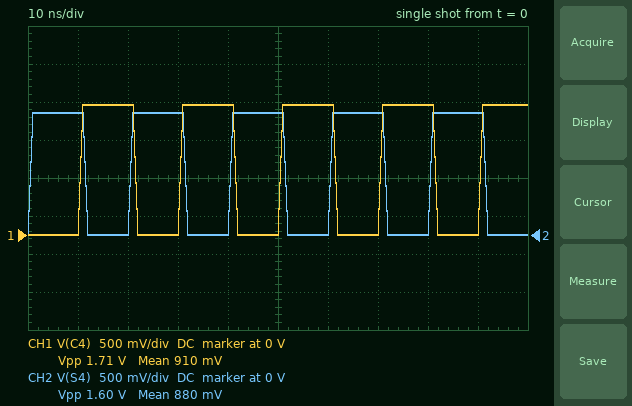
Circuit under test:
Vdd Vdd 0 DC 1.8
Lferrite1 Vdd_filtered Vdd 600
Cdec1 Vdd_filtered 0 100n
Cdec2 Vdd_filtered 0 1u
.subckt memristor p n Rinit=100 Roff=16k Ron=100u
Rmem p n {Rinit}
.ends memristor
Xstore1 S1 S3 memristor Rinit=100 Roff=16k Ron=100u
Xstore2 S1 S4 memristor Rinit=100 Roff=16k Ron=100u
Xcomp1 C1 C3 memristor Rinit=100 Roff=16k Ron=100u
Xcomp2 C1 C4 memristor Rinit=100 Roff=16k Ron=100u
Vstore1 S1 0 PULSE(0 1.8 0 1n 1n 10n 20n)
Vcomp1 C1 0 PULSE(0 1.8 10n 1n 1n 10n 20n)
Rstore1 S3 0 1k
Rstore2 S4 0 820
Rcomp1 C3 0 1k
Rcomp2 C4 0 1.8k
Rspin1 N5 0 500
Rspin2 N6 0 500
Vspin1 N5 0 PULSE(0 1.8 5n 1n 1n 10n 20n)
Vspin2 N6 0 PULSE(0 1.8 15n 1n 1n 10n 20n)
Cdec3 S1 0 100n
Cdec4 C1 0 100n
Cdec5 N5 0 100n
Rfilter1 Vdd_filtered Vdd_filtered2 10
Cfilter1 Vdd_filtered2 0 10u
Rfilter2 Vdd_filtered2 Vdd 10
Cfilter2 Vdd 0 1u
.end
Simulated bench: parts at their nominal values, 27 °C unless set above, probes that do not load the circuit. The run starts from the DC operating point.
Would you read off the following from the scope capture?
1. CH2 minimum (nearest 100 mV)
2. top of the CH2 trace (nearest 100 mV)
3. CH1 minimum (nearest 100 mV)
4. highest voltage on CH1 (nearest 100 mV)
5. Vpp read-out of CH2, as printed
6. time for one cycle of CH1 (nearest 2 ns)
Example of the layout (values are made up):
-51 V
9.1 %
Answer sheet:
0 V
1.6 V
0 V
1.7 V
1.60 V
20 ns
